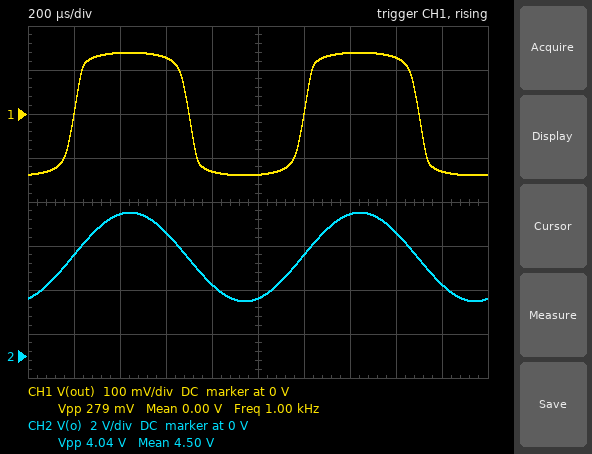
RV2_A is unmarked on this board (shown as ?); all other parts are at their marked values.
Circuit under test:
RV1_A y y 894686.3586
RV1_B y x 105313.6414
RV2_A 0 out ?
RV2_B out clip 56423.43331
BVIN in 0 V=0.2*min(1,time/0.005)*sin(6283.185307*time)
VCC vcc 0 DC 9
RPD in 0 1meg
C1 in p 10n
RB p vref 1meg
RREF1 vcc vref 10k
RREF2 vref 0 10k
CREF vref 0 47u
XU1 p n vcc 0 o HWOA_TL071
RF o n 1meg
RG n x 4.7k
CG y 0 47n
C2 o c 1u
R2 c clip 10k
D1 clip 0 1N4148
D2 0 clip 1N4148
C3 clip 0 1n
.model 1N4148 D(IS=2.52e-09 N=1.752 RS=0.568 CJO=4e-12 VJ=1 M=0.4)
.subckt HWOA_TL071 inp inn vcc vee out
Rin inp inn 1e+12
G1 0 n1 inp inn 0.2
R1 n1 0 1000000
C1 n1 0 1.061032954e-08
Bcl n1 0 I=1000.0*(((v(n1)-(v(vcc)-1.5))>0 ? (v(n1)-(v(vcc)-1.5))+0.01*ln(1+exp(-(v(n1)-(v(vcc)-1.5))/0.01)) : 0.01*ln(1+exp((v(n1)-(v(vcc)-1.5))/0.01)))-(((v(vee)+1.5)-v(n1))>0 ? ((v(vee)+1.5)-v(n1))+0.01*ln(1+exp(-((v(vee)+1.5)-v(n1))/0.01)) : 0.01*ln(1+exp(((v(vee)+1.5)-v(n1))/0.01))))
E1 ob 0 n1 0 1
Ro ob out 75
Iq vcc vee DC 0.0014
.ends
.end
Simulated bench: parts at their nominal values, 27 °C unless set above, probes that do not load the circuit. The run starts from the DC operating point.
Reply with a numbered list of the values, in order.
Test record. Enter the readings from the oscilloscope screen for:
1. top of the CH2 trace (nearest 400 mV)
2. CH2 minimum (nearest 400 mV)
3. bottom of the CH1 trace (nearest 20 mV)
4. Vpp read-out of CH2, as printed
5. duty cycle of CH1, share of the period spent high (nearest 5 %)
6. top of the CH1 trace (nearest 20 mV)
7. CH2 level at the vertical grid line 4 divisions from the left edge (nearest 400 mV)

1. 6.4 V
2. 2.4 V
3. -140 mV
4. 4.04 V
5. 50 %
6. 140 mV
7. 3.2 V
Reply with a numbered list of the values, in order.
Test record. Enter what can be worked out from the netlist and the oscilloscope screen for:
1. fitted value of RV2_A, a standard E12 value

1. 22 kΩ
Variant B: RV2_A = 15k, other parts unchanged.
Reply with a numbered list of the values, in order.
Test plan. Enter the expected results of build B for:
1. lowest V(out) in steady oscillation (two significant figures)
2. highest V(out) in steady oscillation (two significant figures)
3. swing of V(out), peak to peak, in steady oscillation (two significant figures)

1. -100 mV
2. 100 mV
3. 210 mV
